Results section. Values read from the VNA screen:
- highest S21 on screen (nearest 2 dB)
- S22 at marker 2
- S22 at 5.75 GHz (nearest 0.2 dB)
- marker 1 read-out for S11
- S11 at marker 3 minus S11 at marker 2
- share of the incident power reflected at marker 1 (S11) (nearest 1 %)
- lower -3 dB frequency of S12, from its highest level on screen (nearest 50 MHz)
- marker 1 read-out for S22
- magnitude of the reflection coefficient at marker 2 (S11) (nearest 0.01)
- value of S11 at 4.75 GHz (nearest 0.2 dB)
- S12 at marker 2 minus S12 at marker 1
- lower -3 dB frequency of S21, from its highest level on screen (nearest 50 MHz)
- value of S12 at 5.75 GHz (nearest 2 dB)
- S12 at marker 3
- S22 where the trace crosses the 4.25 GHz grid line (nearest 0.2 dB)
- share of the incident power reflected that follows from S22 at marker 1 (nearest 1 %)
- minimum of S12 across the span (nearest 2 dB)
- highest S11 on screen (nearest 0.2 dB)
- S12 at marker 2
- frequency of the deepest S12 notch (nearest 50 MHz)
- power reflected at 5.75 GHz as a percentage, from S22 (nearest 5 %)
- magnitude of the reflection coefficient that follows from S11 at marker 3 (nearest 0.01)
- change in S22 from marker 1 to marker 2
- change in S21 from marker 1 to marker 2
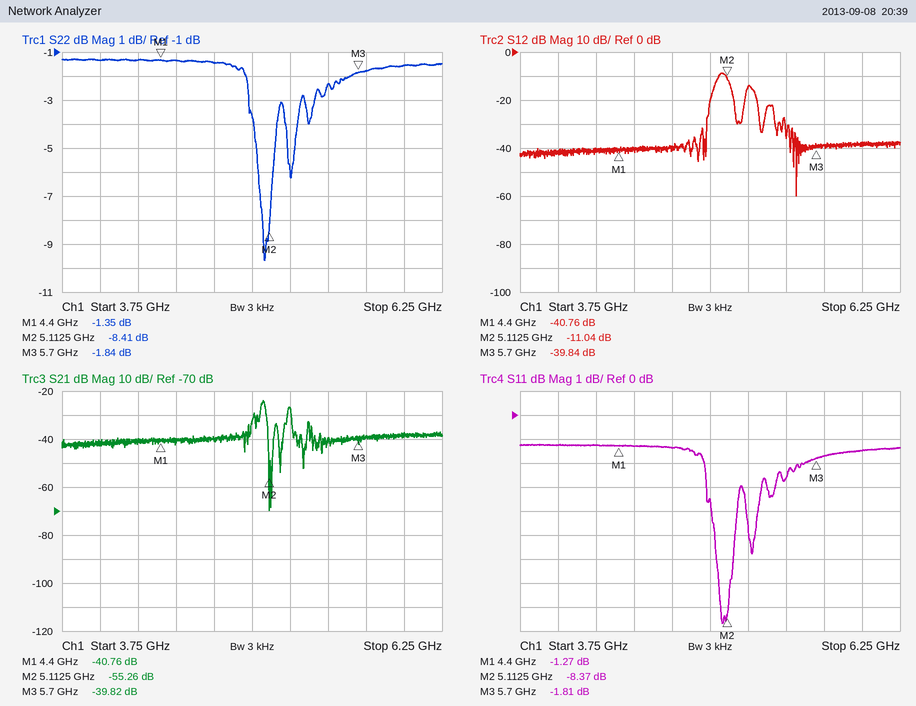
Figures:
-24 dB
-8.41 dB
-1.8 dB
-1.27 dB
6.56 dB
75 %
5.05 GHz
-1.35 dB
0.38
-1.4 dB
29.72 dB
5.05 GHz
-38 dB
-39.84 dB
-1.4 dB
73 %
-60 dB
-1.2 dB
-11.04 dB
5.55 GHz
65 %
0.81
-7.06 dB
-14.50 dB
